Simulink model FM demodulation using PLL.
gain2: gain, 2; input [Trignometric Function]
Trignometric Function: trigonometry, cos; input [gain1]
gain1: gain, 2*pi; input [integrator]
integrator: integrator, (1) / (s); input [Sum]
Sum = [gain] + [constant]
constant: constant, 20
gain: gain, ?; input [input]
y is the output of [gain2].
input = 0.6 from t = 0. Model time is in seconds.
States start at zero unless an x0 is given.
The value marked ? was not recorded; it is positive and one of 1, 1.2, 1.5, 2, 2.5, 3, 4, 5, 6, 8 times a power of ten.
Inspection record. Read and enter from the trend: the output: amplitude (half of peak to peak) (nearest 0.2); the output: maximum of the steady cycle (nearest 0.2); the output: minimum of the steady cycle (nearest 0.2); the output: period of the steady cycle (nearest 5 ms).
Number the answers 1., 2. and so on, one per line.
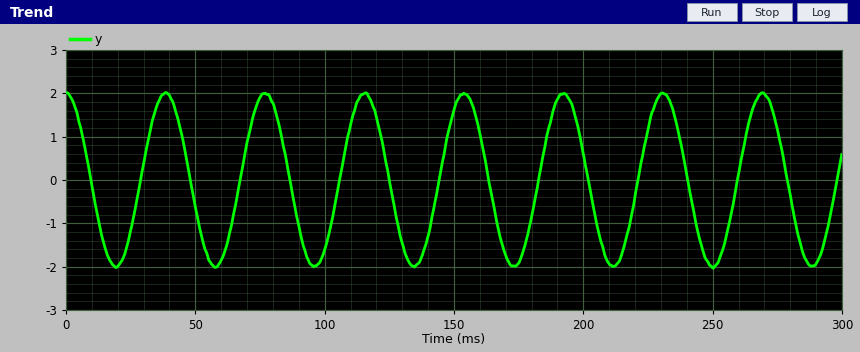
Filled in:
1. 2.0
2. 2.0
3. -2.0
4. 40 ms
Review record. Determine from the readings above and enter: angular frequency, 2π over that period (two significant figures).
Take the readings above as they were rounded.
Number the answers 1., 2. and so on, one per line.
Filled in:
1. 0.16 rad/ms
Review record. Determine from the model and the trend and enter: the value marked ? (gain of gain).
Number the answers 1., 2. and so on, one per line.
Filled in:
1. 10
